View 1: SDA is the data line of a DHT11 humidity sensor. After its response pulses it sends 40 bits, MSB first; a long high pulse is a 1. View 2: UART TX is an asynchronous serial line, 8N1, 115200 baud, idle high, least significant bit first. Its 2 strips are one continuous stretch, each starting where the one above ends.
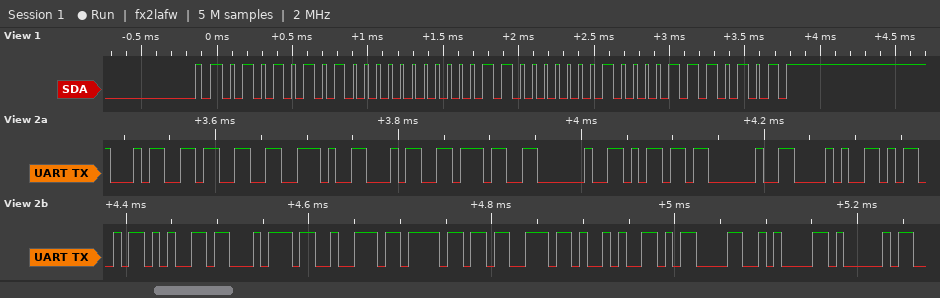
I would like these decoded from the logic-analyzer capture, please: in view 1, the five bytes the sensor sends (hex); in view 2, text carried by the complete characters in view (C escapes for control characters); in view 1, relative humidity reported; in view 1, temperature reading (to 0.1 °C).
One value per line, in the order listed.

55 00 18 08 75
"43.47 m (Metros)\r\nA"
85 %
24.8 °C
